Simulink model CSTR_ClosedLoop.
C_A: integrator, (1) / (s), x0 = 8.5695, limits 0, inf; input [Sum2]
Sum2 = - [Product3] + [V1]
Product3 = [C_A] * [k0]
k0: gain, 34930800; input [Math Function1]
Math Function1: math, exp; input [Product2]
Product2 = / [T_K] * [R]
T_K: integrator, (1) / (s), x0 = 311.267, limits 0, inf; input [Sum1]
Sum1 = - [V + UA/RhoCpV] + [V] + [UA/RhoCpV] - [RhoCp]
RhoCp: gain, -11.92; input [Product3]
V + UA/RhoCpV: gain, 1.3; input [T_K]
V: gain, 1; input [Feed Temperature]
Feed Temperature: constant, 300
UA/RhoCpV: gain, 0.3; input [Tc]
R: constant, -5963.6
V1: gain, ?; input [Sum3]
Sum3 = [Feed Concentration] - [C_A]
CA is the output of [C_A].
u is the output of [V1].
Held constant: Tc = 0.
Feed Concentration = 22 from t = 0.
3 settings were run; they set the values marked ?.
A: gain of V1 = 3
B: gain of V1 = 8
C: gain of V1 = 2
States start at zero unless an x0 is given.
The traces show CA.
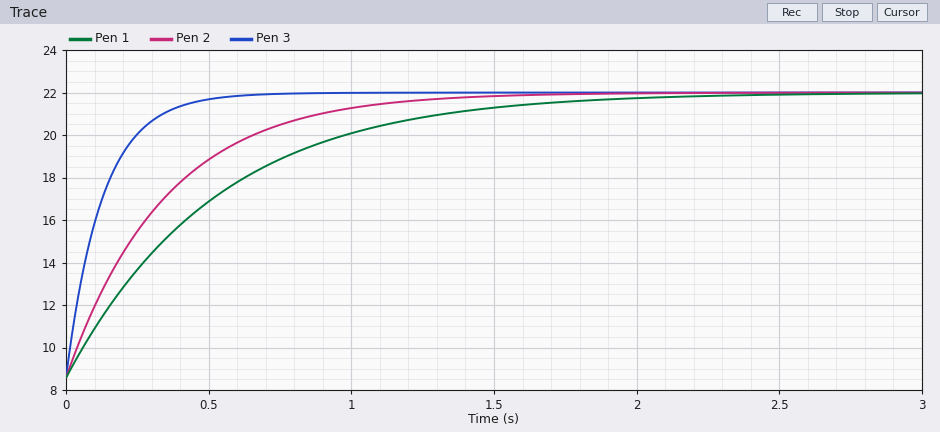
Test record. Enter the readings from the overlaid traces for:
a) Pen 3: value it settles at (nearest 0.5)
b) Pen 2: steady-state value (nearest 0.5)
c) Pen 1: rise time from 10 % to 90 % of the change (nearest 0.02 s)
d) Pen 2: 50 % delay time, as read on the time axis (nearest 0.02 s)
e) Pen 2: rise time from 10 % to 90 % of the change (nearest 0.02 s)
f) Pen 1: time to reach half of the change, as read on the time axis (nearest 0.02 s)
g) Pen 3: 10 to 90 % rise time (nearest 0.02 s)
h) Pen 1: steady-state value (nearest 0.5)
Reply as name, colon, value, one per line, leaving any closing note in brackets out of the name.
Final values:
Pen 3: value it settles at: 22.0
Pen 2: steady-state value: 22.0
Pen 1: rise time from 10 % to 90 % of the change: 1.12 s
Pen 2: 50 % delay time, as read on the time axis: 0.24 s
Pen 2: rise time from 10 % to 90 % of the change: 0.76 s
Pen 1: time to reach half of the change, as read on the time axis: 0.36 s
Pen 3: 10 to 90 % rise time: 0.28 s
Pen 1: steady-state value: 22.0
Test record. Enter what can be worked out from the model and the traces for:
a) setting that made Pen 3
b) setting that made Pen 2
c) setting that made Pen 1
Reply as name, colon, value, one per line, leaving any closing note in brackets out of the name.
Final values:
setting that made Pen 3: B
setting that made Pen 2: A
setting that made Pen 1: C
